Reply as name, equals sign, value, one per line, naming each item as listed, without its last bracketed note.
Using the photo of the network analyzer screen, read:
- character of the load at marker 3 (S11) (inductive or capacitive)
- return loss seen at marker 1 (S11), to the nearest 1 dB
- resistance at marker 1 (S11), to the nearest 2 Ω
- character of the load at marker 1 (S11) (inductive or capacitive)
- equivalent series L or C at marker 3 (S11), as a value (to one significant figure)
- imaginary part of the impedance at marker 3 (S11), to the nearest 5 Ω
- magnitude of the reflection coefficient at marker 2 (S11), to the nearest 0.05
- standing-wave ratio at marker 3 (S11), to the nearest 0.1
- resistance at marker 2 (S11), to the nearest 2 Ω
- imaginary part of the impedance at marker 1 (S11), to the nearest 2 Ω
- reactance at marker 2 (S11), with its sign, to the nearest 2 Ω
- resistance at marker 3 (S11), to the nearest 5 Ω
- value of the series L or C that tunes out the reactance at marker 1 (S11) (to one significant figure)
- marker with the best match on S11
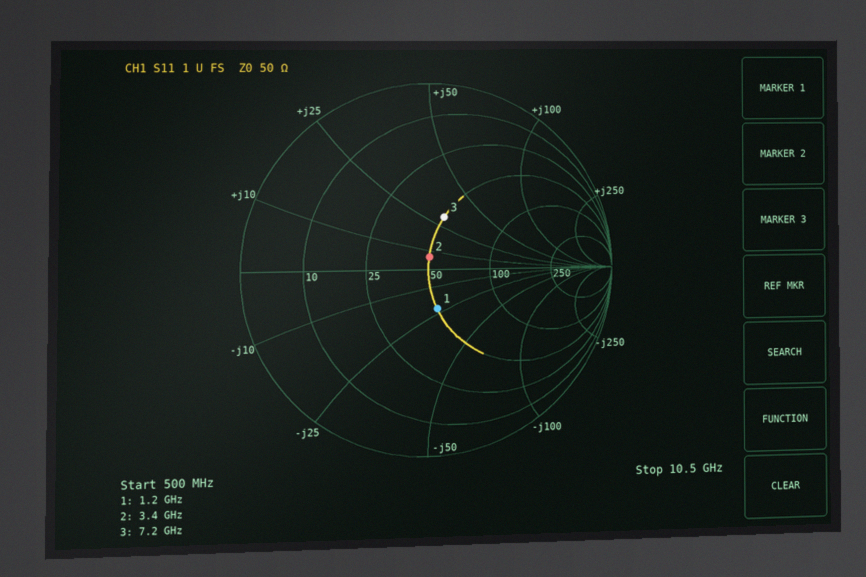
character of the load at marker 3 (S11) = inductive
return loss seen at marker 1 (S11), to the nearest 1 dB = 13 dB
resistance at marker 1 (S11), to the nearest 2 Ω = 50 Ω
character of the load at marker 1 (S11) = capacitive
equivalent series L or C at marker 3 (S11), as a value = 700 pH
imaginary part of the impedance at marker 3 (S11), to the nearest 5 Ω = +30 Ω
magnitude of the reflection coefficient at marker 2 (S11), to the nearest 0.05 = 0.05
standing-wave ratio at marker 3 (S11), to the nearest 0.1 = 1.8
resistance at marker 2 (S11), to the nearest 2 Ω = 50 Ω
imaginary part of the impedance at marker 1 (S11), to the nearest 2 Ω = -22 Ω
reactance at marker 2 (S11), with its sign, to the nearest 2 Ω = +6 Ω
resistance at marker 3 (S11), to the nearest 5 Ω = 50 Ω
value of the series L or C that tunes out the reactance at marker 1 (S11) = 3 nH
marker with the best match on S11 = marker 2
